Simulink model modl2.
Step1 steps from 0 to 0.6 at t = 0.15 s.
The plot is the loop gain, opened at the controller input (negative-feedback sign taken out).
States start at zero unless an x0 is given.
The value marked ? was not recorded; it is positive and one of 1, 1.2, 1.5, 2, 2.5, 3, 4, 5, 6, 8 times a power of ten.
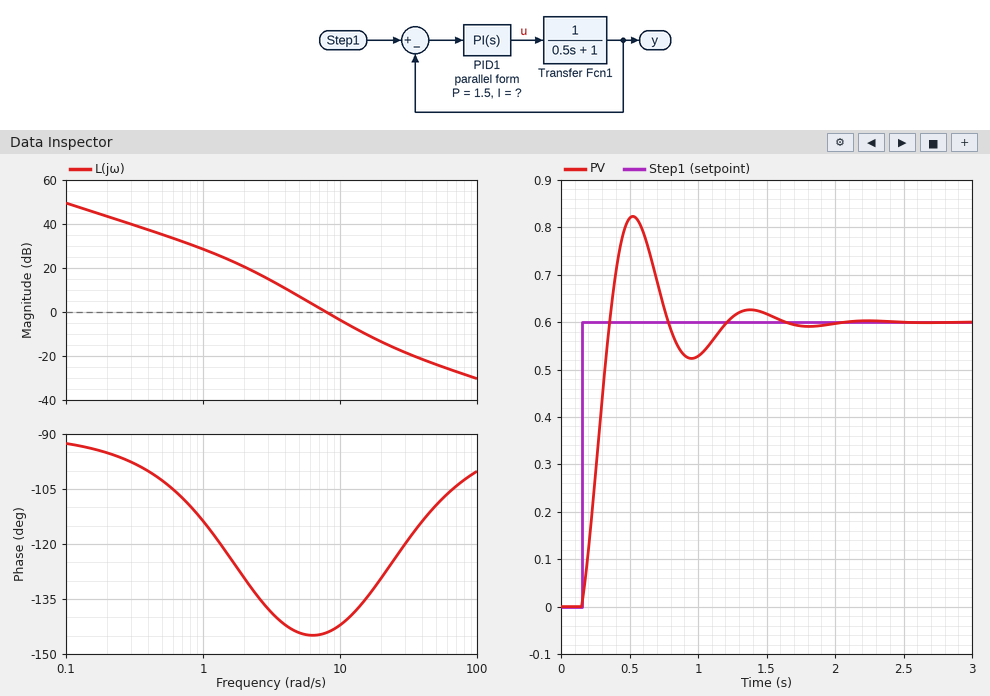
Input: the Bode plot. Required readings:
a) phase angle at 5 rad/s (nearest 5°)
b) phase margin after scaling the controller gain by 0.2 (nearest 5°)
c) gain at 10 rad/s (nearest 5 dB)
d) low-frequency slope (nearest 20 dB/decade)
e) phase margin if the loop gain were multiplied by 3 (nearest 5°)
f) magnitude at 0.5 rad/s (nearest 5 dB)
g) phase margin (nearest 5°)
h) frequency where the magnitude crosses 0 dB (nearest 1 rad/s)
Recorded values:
-145°
40°
-5 dB
-20 dB/decade
45°
35 dB
35°
8 rad/s
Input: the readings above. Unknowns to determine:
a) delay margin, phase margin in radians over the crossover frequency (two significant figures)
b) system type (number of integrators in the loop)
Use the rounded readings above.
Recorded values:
0.076 s
1
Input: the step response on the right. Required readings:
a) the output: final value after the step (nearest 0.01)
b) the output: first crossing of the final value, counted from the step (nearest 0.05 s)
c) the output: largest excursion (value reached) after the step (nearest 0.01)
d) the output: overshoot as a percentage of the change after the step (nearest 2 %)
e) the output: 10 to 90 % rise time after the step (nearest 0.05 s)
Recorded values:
0.60
0.20 s
0.82
38 %
0.15 s
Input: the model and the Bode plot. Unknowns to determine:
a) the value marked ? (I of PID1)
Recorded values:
30
